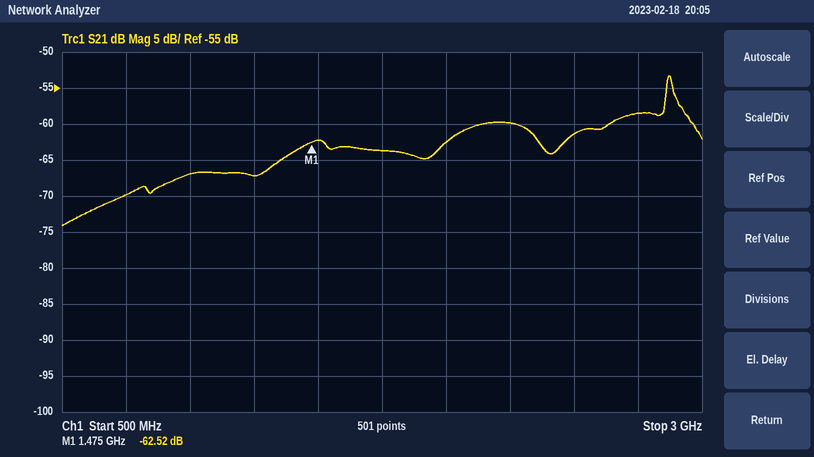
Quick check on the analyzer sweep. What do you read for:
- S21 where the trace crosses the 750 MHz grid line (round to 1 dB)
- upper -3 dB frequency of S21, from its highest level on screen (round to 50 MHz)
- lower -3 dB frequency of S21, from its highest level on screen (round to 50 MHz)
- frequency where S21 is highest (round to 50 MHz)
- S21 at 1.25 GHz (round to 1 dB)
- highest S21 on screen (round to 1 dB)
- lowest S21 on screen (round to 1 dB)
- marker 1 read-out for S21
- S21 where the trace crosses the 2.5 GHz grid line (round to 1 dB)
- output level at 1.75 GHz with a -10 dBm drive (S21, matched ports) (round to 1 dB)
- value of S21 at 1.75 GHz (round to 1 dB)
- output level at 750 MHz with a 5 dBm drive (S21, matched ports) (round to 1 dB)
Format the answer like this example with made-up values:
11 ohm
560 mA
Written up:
-70 dB
2.90 GHz
2.85 GHz
2.85 GHz
-67 dB
-53 dB
-74 dB
-62.52 dB
-61 dB
-74 dBm
-64 dB
-65 dBm
